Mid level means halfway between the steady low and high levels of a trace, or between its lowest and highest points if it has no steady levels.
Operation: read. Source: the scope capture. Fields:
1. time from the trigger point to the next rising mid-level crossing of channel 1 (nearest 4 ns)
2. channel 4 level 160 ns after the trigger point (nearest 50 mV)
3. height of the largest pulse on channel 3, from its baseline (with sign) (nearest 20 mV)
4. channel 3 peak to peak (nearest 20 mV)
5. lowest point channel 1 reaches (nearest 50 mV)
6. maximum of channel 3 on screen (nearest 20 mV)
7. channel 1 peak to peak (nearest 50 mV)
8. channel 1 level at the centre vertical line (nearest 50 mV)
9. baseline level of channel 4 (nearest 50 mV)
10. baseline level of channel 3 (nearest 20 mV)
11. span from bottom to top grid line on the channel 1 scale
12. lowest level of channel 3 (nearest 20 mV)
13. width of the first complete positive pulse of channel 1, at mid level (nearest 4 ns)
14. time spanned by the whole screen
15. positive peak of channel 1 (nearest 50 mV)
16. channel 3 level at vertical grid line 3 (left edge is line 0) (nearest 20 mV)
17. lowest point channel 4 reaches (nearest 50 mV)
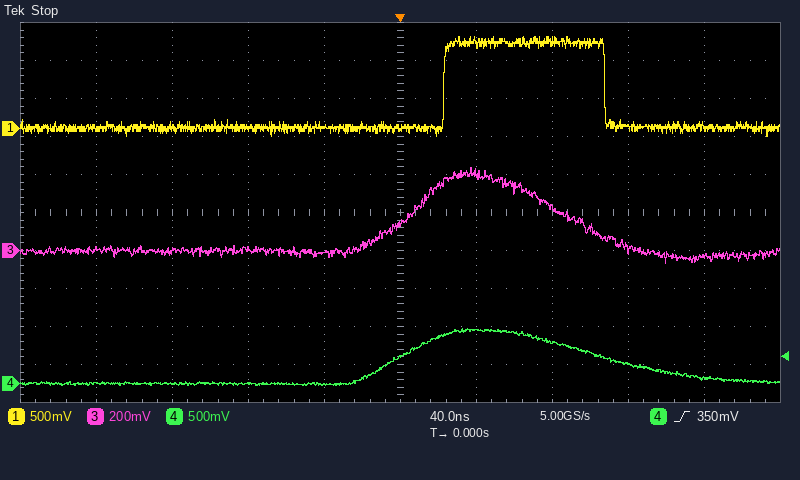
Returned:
24 ns
50 mV
+440 mV
500 mV
-100 mV
440 mV
1.30 V
0 mV
0 mV
0 mV
5 V
-60 mV
84 ns
400 ns
1.20 V
0 mV
-50 mV
